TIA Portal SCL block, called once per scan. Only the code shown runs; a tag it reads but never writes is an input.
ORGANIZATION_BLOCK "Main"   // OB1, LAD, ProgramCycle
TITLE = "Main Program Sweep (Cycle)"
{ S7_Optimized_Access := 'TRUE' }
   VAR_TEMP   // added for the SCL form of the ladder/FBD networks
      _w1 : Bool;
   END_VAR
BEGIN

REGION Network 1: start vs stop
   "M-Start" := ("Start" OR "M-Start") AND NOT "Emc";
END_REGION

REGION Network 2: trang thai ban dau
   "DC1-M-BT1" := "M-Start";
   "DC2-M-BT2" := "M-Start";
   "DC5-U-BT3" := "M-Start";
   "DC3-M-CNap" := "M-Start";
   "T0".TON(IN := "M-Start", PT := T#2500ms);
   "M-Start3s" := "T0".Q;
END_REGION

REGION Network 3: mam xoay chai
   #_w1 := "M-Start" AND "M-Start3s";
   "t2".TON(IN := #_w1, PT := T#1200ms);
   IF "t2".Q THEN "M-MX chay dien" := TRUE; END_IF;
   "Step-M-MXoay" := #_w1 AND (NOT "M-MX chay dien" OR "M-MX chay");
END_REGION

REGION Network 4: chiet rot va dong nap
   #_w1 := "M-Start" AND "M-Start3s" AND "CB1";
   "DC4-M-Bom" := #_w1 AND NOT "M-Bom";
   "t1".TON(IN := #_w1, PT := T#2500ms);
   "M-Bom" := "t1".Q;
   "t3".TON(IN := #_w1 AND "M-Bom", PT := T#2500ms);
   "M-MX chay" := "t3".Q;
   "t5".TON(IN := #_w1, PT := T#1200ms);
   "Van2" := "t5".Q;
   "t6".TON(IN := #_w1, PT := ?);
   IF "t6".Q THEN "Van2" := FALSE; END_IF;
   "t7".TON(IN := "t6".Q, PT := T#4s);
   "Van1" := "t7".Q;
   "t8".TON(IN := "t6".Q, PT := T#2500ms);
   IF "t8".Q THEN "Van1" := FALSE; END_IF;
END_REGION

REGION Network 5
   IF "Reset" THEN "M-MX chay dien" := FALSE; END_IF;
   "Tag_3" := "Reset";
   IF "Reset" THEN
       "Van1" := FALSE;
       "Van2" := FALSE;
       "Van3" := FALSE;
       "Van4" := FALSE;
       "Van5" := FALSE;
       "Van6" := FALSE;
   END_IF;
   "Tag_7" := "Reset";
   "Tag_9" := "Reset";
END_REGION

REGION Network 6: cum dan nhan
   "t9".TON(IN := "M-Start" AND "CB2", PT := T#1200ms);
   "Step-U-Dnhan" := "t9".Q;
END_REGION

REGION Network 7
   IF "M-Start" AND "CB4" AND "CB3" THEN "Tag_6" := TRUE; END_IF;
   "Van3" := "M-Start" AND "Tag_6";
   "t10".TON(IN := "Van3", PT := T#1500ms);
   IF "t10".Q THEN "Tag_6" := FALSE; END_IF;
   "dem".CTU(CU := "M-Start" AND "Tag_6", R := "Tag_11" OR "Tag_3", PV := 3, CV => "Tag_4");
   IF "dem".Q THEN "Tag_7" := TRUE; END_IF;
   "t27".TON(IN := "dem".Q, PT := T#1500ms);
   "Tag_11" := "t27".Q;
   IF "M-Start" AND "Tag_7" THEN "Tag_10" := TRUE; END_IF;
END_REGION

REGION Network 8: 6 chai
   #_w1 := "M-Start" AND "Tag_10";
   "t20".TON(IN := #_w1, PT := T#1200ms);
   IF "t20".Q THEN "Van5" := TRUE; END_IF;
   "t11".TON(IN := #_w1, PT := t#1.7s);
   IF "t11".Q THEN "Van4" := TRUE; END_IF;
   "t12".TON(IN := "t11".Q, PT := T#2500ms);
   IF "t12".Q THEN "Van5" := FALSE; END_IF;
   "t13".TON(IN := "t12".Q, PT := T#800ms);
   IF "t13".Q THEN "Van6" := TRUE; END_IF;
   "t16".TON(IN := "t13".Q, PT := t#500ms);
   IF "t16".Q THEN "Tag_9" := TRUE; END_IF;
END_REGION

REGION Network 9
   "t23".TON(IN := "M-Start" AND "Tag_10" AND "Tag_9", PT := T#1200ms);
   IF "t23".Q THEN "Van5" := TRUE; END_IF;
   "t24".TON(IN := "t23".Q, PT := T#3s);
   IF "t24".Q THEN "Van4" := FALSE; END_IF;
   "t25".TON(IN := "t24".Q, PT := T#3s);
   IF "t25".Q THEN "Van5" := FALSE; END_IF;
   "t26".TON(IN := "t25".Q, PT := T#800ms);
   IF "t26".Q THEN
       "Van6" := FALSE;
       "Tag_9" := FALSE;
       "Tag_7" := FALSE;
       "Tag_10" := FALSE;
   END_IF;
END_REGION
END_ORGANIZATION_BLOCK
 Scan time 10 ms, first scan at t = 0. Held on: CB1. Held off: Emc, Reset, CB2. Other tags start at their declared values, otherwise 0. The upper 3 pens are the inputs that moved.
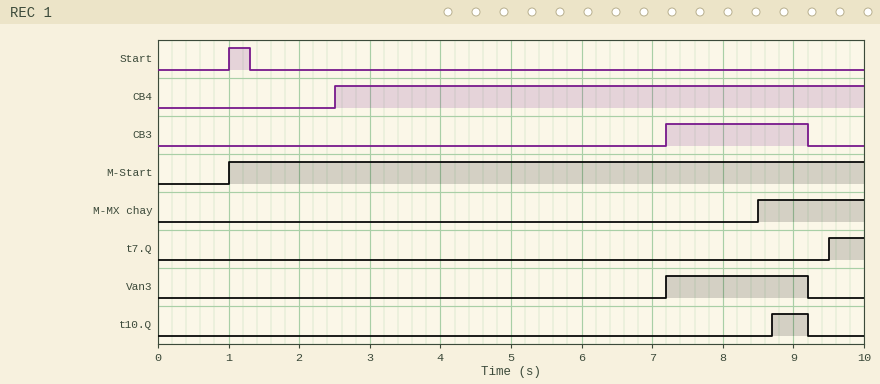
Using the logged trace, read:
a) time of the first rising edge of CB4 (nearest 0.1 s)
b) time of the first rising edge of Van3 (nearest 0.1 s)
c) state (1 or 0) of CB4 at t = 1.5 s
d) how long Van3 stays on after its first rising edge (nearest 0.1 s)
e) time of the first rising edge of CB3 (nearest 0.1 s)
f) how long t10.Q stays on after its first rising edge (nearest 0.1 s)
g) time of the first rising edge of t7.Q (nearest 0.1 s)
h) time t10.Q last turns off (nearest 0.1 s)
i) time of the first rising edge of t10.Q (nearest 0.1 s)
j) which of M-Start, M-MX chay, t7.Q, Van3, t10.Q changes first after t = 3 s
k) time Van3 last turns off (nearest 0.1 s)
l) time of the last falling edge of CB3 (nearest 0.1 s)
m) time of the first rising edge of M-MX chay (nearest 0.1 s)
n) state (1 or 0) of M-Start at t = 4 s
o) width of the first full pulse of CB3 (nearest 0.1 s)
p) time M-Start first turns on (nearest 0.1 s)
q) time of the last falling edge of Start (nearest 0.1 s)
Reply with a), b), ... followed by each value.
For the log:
a) 2.5 s
b) 7.2 s
c) 0
d) 2.0 s
e) 7.2 s
f) 0.5 s
g) 9.5 s
h) 9.2 s
i) 8.7 s
j) Van3
k) 9.2 s
l) 9.2 s
m) 8.5 s
n) 1
o) 2.0 s
p) 1.0 s
q) 1.3 s
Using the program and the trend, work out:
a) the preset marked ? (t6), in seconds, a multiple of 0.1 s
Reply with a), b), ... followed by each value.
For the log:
a) 2.0 s
